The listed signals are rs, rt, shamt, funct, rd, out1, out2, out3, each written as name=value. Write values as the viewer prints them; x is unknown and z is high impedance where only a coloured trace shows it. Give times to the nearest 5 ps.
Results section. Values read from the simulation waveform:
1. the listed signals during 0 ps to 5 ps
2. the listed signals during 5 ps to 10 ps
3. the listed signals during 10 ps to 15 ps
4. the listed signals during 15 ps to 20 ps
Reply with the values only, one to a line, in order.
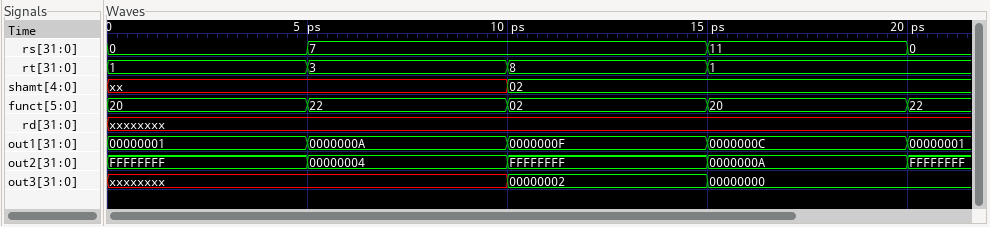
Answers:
rs=0, rt=1, shamt=xx, funct=20, rd=xxxxxxxx, out1=00000001, out2=FFFFFFFF, out3=xxxxxxxx
rs=7, rt=3, shamt=xx, funct=22, rd=xxxxxxxx, out1=0000000A, out2=00000004, out3=xxxxxxxx
rs=7, rt=8, shamt=02, funct=02, rd=xxxxxxxx, out1=0000000F, out2=FFFFFFFF, out3=00000002
rs=11, rt=1, shamt=02, funct=20, rd=xxxxxxxx, out1=0000000C, out2=0000000A, out3=00000000
